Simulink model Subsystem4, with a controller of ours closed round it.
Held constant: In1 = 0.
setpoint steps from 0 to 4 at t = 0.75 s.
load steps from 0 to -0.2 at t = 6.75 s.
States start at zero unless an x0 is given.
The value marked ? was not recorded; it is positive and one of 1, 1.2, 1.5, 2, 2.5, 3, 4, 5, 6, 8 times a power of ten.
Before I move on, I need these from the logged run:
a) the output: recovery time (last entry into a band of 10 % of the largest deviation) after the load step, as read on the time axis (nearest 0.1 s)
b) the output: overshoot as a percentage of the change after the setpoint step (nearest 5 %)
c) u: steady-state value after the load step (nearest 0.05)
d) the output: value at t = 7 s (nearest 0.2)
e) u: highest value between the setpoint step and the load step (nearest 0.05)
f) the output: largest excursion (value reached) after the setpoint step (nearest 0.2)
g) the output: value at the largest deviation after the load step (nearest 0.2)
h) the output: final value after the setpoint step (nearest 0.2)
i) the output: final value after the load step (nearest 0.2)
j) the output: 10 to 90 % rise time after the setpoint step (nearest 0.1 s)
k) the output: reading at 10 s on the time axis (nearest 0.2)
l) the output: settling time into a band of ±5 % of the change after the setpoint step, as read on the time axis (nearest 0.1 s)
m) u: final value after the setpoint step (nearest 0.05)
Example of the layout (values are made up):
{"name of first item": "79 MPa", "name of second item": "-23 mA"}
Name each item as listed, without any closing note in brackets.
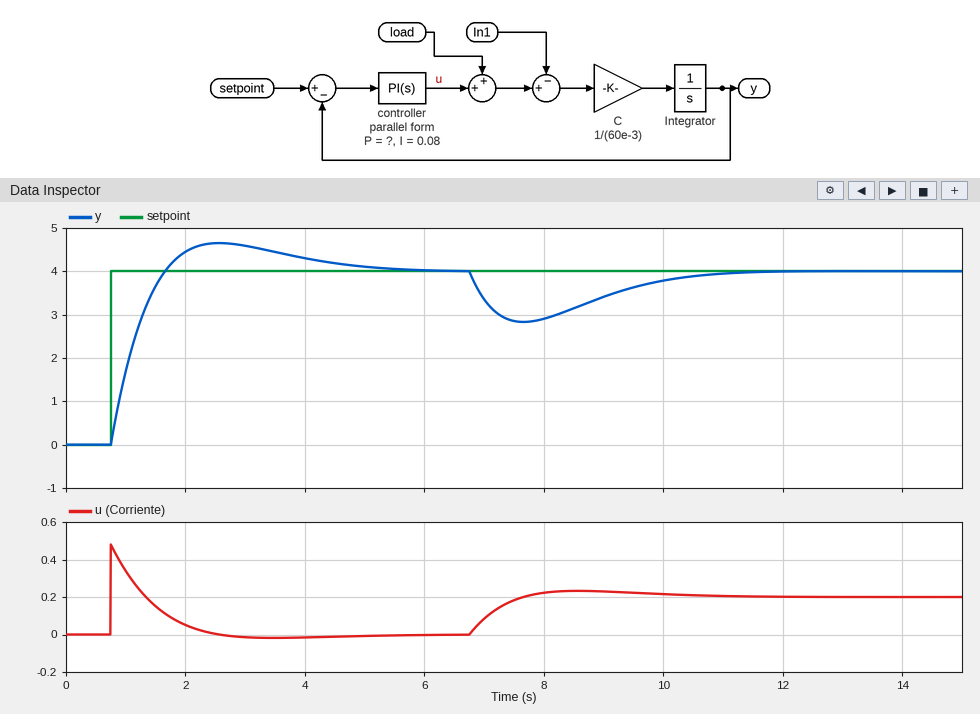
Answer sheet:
{"the output: recovery time (last entry into a band of 10 % of the largest deviation) after the load step, as read on the time axis": "10.5 s", "the output: overshoot as a percentage of the change after the setpoint step": "15 %", "u: steady-state value after the load step": "0.20", "the output: value at t = 7 s": "3.4", "u: highest value between the setpoint step and the load step": "0.50", "the output: largest excursion (value reached) after the setpoint step": "4.6", "the output: value at the largest deviation after the load step": "2.8", "the output: final value after the setpoint step": "4.0", "the output: final value after the load step": "4.0", "the output: 10 to 90 % rise time after the setpoint step": "0.7 s", "the output: reading at 10 s on the time axis": "3.8", "the output: settling time into a band of ±5 % of the change after the setpoint step, as read on the time axis": "4.4 s", "u: final value after the setpoint step": "0.00"}
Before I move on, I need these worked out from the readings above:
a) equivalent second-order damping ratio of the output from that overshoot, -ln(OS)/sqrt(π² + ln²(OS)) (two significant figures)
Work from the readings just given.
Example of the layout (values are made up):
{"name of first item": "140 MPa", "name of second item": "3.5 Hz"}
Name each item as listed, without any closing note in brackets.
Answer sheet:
{"equivalent second-order damping ratio of the output from that overshoot, -ln(OS)/sqrt(π² + ln²(OS))": "0.52"}
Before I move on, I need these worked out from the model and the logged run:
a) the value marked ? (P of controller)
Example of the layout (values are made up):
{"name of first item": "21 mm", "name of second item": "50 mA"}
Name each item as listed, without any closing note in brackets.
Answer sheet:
{"the value marked ?": "0.12"}
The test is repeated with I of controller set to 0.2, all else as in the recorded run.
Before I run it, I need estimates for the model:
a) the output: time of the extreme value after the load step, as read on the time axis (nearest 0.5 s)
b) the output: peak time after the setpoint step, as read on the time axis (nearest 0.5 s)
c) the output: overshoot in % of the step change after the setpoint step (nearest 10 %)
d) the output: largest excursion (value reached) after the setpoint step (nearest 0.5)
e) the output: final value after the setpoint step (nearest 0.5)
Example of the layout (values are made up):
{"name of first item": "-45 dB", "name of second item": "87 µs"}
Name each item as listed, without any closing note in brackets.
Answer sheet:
{"the output: time of the extreme value after the load step, as read on the time axis": "7.5 s", "the output: peak time after the setpoint step, as read on the time axis": "2.0 s", "the output: overshoot in % of the step change after the setpoint step": "30 %", "the output: largest excursion (value reached) after the setpoint step": "5.0", "the output: final value after the setpoint step": "4.0"}
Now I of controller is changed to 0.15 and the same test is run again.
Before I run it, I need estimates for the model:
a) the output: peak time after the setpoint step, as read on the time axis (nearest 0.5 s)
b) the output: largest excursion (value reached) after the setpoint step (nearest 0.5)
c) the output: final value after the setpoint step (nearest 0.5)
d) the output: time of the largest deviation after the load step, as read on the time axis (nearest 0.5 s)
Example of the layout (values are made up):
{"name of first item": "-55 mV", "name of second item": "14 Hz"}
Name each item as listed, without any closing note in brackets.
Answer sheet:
{"the output: peak time after the setpoint step, as read on the time axis": "2.0 s", "the output: largest excursion (value reached) after the setpoint step": "5.0", "the output: final value after the setpoint step": "4.0", "the output: time of the largest deviation after the load step, as read on the time axis": "7.5 s"}
